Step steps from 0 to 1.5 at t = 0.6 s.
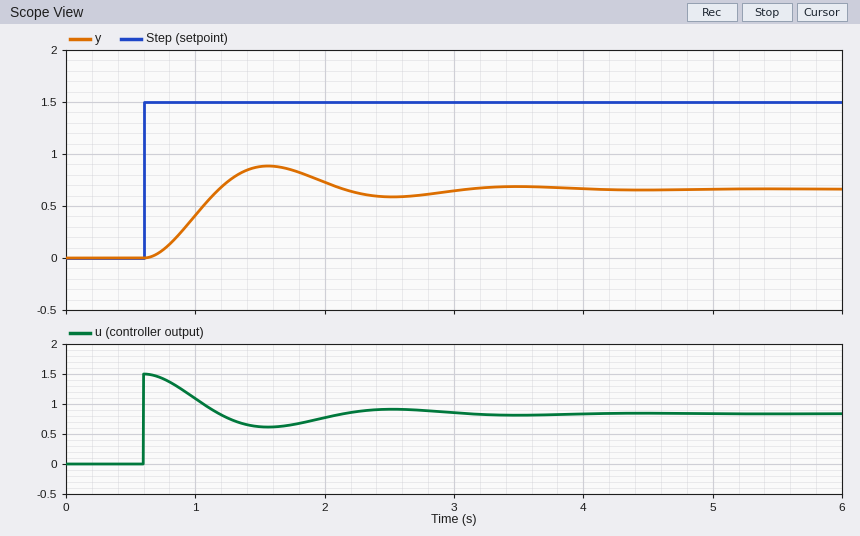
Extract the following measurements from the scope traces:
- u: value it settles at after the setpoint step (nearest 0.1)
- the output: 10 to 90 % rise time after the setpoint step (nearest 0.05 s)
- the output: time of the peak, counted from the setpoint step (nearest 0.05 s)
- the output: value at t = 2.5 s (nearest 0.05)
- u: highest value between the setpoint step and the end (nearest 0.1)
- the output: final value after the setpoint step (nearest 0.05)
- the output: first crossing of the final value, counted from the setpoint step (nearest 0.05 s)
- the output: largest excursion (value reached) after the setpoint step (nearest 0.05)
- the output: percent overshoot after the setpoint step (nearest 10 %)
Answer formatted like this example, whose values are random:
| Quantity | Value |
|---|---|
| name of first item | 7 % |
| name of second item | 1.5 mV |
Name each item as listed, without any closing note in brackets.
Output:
| Quantity | Value |
|---|---|
| u: value it settles at after the setpoint step | 0.8 |
| the output: 10 to 90 % rise time after the setpoint step | 0.40 s |
| the output: time of the peak, counted from the setpoint step | 0.95 s |
| the output: value at t = 2.5 s | 0.60 |
| u: highest value between the setpoint step and the end | 1.5 |
| the output: final value after the setpoint step | 0.65 |
| the output: first crossing of the final value, counted from the setpoint step | 0.60 s |
| the output: largest excursion (value reached) after the setpoint step | 0.90 |
| the output: percent overshoot after the setpoint step | 30 % |
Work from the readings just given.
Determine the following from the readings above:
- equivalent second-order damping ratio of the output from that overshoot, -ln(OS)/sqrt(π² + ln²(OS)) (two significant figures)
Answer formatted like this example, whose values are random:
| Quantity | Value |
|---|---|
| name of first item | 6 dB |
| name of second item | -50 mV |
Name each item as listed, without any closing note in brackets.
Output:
| Quantity | Value |
|---|---|
| equivalent second-order damping ratio of the output from that overshoot, -ln(OS)/sqrt(π² + ln²(OS)) | 0.36 |
